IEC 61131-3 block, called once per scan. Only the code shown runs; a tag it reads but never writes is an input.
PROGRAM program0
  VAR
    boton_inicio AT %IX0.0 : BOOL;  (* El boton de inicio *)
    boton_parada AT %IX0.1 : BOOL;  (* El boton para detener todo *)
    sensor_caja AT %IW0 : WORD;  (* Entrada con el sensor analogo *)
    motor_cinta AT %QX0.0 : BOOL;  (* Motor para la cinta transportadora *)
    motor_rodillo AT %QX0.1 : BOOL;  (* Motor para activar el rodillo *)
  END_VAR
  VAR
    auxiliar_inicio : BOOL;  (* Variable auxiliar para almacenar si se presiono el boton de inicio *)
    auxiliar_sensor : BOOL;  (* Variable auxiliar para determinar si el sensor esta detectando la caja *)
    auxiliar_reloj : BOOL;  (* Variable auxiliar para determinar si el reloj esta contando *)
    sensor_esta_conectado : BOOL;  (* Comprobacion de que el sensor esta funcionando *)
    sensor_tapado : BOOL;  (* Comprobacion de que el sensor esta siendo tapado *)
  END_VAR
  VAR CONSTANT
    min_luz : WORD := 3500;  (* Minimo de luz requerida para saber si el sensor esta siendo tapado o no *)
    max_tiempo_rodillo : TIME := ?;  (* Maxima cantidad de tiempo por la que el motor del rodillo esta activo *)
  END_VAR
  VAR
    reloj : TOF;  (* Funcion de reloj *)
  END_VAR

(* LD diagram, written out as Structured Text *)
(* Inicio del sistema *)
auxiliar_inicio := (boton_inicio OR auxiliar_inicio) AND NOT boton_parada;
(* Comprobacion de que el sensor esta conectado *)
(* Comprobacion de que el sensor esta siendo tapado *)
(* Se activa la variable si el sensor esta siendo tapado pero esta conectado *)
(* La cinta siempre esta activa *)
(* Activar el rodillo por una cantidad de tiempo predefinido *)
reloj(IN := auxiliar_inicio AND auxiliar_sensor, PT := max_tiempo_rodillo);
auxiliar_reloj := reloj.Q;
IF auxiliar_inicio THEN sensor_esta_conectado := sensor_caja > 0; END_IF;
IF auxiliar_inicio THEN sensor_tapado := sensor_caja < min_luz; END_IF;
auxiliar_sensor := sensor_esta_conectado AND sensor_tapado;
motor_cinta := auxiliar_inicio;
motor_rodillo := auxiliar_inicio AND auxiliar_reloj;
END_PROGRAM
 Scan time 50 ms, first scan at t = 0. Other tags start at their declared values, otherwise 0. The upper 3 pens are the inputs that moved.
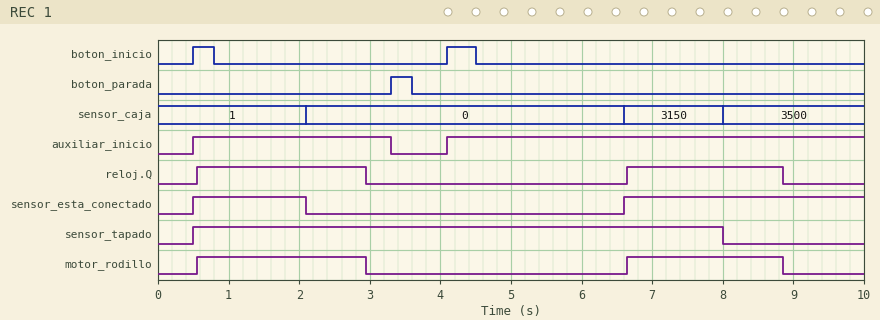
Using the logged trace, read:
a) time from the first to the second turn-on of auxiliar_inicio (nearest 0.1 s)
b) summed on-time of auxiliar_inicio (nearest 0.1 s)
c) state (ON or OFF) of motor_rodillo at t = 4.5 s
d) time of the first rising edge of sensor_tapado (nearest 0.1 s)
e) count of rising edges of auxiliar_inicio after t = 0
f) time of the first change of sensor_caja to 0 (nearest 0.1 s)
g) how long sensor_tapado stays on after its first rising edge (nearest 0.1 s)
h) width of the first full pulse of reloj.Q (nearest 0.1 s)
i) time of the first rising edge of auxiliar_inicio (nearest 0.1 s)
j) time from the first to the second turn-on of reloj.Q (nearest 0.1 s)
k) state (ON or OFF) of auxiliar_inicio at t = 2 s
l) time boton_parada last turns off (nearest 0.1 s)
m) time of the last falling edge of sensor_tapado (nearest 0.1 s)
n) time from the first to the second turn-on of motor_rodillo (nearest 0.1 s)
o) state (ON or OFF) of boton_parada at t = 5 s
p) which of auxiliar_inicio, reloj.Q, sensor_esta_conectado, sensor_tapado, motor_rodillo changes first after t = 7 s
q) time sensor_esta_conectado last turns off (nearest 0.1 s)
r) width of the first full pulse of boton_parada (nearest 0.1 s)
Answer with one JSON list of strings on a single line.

["3.6 s", "8.7 s", "OFF", "0.5 s", "2", "2.1 s", "7.5 s", "2.4 s", "0.5 s", "6.1 s", "ON", "3.6 s", "8.0 s", "6.1 s", "OFF", "sensor_tapado", "2.1 s", "0.3 s"]
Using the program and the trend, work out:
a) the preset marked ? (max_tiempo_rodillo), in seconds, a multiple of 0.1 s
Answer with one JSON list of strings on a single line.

["0.8 s"]
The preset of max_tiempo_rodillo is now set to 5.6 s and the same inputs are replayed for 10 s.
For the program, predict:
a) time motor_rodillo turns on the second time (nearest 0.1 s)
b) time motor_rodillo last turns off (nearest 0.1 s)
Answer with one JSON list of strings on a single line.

["4.1 s", "3.3 s"]
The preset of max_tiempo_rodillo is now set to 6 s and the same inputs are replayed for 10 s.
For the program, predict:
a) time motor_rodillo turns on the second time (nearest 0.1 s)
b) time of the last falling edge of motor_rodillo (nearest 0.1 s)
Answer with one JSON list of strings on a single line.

["4.1 s", "3.3 s"]
